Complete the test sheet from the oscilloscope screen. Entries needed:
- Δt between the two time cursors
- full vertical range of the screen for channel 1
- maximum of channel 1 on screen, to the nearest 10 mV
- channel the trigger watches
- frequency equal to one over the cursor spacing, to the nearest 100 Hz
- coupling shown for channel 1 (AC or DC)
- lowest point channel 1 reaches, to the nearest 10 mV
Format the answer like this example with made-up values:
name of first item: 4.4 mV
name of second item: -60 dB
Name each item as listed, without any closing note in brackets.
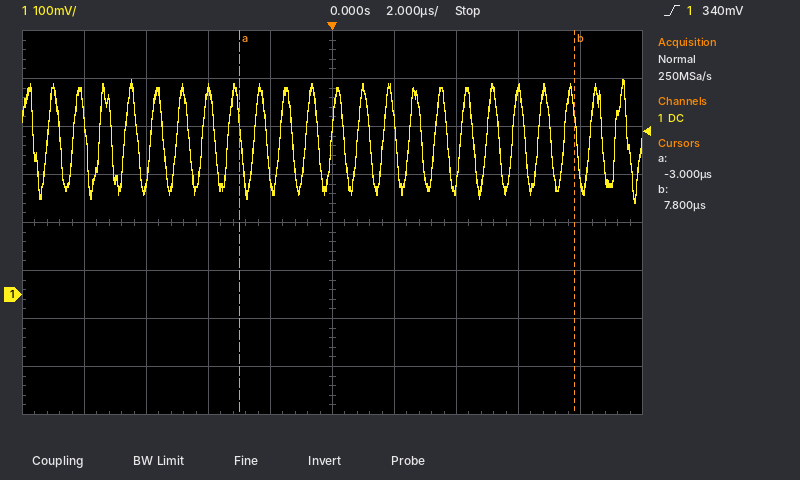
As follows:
Δt between the two time cursors: 10.8 µs
full vertical range of the screen for channel 1: 800 mV
maximum of channel 1 on screen, to the nearest 10 mV: 450 mV
channel the trigger watches: channel 1
frequency equal to one over the cursor spacing, to the nearest 100 Hz: 92.6 kHz
coupling shown for channel 1: DC
lowest point channel 1 reaches, to the nearest 10 mV: 190 mV
